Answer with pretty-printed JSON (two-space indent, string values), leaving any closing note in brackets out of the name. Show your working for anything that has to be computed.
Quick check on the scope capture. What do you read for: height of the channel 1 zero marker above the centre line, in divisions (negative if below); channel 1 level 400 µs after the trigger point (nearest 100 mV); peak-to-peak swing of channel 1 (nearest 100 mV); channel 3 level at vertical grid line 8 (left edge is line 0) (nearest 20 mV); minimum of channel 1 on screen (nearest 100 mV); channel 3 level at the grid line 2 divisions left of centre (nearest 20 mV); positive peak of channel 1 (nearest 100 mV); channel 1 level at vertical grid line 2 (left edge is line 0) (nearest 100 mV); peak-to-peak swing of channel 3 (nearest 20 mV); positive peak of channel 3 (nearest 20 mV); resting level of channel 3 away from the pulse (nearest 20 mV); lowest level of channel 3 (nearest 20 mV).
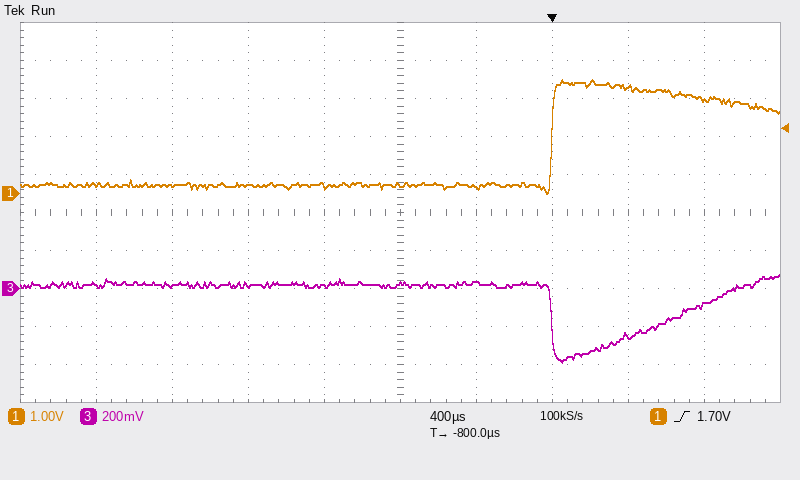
{
  "height of the channel 1 zero marker above the centre line, in divisions": "+0.5 div",
  "channel 1 level 400 µs after the trigger point": "2.8 V",
  "peak-to-peak swing of channel 1": "3.0 V − (0.0 V) = 3.0 V",
  "channel 3 level at vertical grid line 8 (left edge is line 0)": "-240 mV",
  "minimum of channel 1 on screen": "0.0 V",
  "channel 3 level at the grid line 2 divisions left of centre": "20 mV",
  "positive peak of channel 1": "3.0 V",
  "channel 1 level at vertical grid line 2 (left edge is line 0)": "200 mV",
  "peak-to-peak swing of channel 3": "80 mV − (-380 mV) = 460 mV",
  "positive peak of channel 3": "80 mV",
  "resting level of channel 3 away from the pulse": "20 mV",
  "lowest level of channel 3": "-380 mV"
}
